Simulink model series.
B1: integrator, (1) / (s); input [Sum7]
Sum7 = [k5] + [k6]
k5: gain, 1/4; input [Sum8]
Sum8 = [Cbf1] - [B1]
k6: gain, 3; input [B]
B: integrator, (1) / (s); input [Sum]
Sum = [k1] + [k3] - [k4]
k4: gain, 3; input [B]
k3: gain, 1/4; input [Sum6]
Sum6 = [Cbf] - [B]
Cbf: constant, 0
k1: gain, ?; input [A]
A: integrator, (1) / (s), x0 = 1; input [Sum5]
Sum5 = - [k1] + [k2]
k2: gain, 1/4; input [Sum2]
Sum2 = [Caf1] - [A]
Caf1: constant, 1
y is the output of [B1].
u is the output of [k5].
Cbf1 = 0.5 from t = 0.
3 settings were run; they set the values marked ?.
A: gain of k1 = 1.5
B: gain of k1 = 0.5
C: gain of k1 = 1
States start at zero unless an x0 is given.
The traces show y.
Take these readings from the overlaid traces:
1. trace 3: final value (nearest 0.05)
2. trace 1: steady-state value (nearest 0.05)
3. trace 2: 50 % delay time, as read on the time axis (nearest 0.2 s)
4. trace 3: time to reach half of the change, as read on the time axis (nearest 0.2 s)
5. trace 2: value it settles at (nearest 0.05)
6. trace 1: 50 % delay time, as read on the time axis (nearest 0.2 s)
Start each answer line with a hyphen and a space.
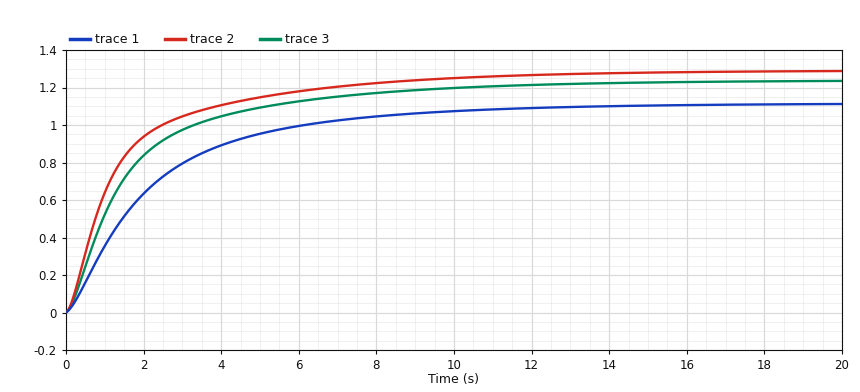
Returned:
- 1.25
- 1.10
- 1.0 s
- 1.2 s
- 1.30
- 1.6 s
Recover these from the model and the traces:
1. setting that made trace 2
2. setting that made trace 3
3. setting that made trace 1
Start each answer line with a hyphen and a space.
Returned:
- A
- C
- B
